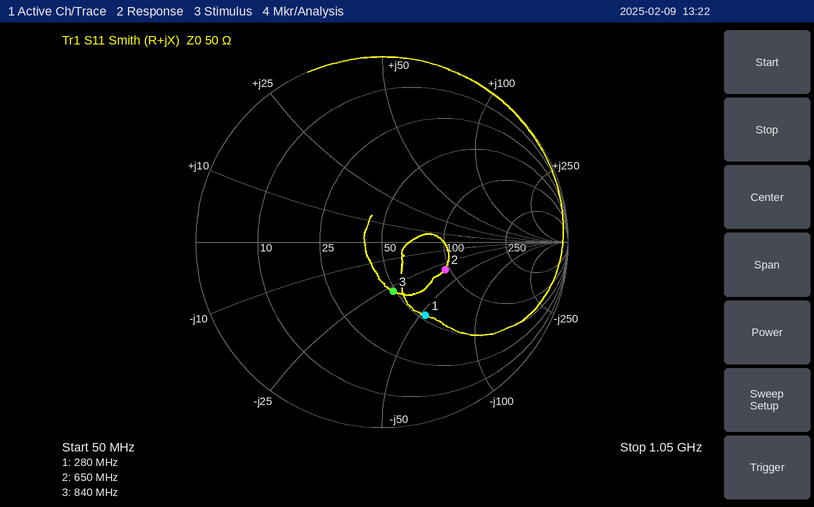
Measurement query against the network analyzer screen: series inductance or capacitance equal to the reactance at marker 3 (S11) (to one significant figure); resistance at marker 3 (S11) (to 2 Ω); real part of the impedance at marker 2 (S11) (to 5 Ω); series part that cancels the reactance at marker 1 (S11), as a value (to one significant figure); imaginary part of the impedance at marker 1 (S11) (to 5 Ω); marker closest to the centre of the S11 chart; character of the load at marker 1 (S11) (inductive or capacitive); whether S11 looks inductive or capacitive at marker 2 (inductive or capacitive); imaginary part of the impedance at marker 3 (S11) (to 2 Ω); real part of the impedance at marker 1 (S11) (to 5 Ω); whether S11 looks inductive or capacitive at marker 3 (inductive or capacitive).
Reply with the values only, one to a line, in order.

7 pF
48 Ω
95 Ω
30 nH
-55 Ω
marker 3
capacitive
capacitive
-28 Ω
55 Ω
capacitive
